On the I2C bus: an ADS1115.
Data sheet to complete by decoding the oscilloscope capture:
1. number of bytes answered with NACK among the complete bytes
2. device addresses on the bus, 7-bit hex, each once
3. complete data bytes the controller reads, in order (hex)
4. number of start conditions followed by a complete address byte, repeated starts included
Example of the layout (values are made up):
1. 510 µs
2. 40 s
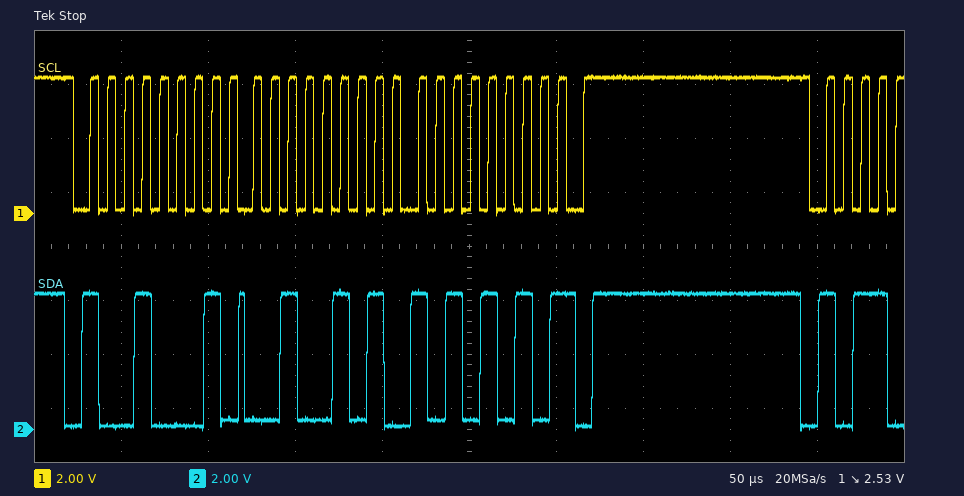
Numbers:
1. 1
2. 0x48
3. 25 AA
4. 1
